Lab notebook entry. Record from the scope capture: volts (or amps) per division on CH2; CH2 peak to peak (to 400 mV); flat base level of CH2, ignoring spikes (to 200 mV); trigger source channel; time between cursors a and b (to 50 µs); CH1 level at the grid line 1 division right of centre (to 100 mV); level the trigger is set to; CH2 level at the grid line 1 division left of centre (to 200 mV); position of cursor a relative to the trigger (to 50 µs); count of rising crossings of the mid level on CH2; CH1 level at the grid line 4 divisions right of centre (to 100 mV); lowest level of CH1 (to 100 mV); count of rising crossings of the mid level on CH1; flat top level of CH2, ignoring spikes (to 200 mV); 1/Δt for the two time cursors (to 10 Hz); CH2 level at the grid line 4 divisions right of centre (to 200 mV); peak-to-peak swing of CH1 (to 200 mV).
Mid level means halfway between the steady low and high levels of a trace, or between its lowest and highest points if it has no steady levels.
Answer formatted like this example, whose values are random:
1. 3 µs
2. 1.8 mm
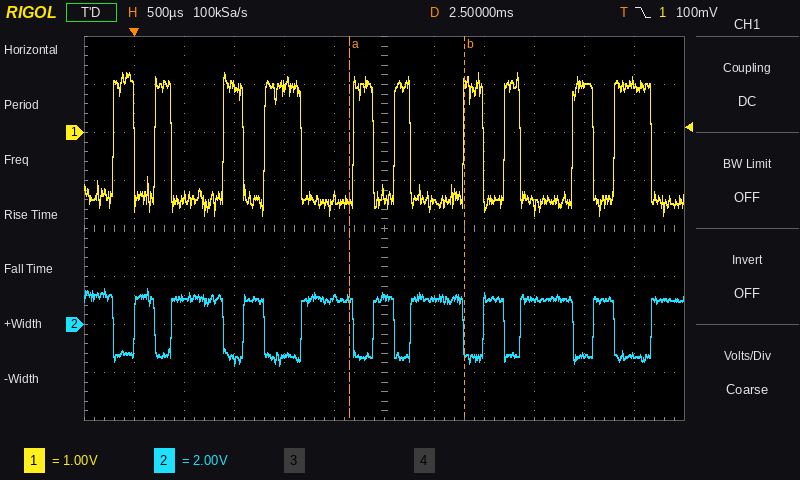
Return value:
1. 2 V
2. 3.2 V
3. -1.4 V
4. CH1
5. 1.15 ms
6. -1.4 V
7. 100 mV
8. 1.2 V
9. +2.15 ms
10. 10
11. 1.0 V
12. -1.7 V
13. 10
14. 1.0 V
15. 870 Hz
16. -1.2 V
17. 3.0 V
